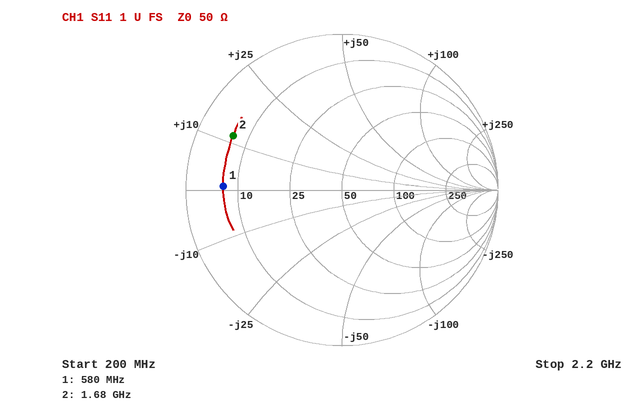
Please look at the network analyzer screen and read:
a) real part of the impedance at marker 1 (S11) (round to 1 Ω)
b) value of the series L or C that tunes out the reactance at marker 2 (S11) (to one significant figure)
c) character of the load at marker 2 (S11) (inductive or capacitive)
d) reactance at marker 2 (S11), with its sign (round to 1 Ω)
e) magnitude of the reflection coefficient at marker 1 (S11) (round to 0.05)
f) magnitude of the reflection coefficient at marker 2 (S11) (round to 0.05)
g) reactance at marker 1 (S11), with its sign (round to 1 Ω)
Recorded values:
7 Ω
8 pF
inductive
+12 Ω
0.75
0.80
+1 Ω
